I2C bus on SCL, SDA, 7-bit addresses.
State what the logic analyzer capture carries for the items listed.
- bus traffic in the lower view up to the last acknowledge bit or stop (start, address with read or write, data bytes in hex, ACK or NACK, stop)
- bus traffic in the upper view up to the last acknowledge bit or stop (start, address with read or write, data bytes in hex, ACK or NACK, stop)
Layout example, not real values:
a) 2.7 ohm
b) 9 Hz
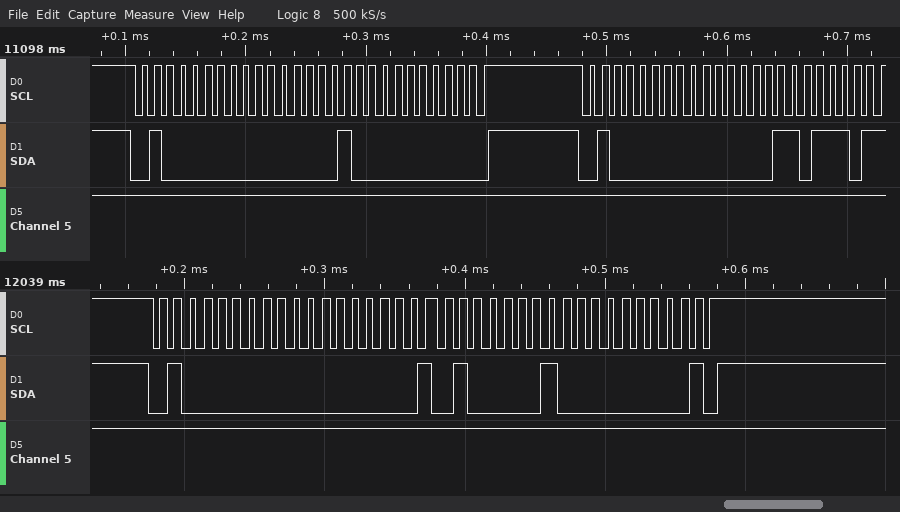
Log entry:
a) start, address 20 write ACK, 00 ACK, repeated start, address 20 read ACK, 00 NACK, stop
b) start, address 20 write ACK, 01 ACK, 00 ACK, stop, start, address 20 write ACK, 03 ACK
